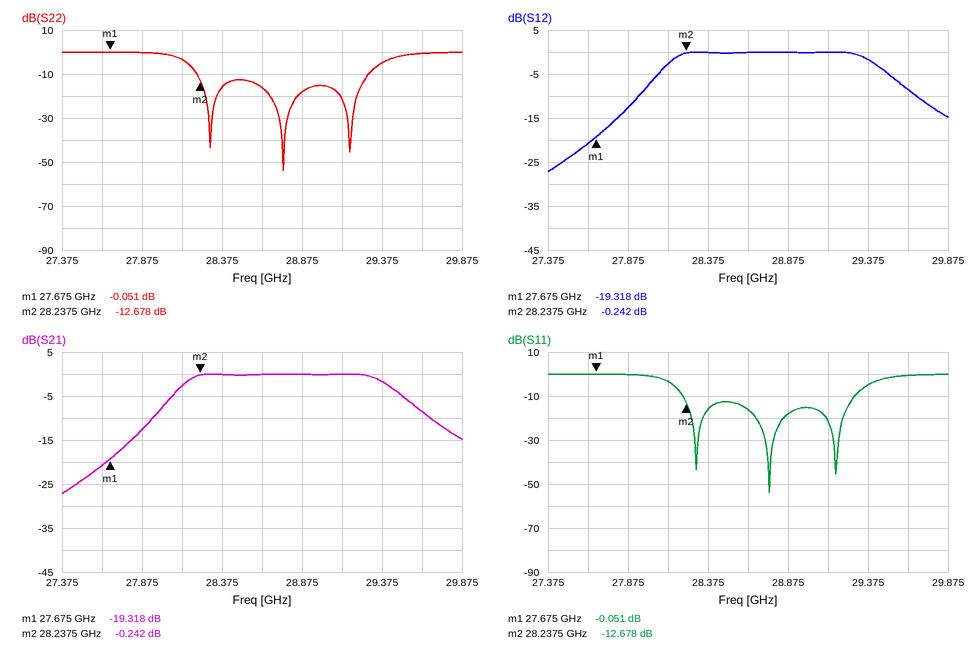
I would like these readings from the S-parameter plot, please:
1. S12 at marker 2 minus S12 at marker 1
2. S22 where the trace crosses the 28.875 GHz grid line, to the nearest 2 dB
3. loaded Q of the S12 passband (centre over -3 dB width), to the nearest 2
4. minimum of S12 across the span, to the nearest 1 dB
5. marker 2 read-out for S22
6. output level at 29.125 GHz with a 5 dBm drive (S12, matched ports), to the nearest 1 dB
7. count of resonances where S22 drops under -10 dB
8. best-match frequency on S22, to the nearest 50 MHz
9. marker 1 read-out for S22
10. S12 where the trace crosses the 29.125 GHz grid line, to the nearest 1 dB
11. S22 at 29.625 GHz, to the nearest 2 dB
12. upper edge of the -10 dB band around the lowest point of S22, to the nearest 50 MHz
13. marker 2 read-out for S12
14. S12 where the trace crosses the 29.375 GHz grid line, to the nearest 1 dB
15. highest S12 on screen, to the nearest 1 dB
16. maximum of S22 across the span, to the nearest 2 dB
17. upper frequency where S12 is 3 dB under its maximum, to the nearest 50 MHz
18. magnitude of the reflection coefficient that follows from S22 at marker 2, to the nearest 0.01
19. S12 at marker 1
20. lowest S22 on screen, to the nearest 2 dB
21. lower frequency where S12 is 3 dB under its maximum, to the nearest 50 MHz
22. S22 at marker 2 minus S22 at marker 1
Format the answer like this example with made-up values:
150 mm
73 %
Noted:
19.076 dB
-18 dB
22
-27 dB
-12.678 dB
5 dBm
3
28.75 GHz
-0.051 dB
0 dB
0 dB
29.30 GHz
-0.242 dB
-2 dB
0 dB
0 dB
29.45 GHz
0.23
-19.318 dB
-54 dB
28.10 GHz
-12.627 dB
